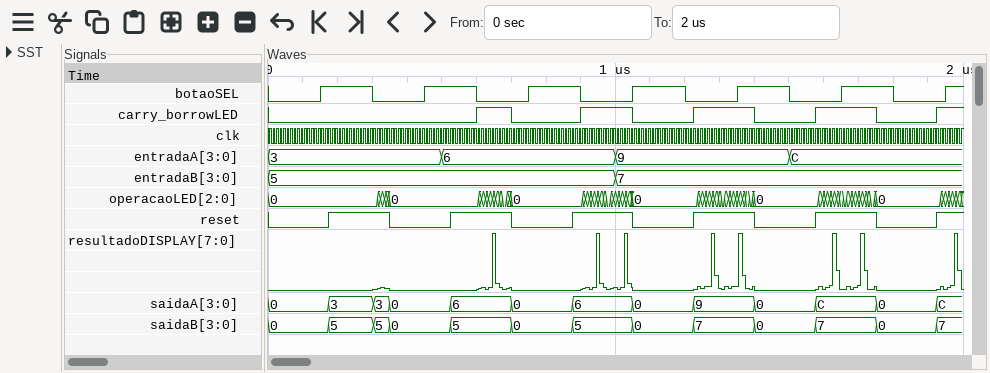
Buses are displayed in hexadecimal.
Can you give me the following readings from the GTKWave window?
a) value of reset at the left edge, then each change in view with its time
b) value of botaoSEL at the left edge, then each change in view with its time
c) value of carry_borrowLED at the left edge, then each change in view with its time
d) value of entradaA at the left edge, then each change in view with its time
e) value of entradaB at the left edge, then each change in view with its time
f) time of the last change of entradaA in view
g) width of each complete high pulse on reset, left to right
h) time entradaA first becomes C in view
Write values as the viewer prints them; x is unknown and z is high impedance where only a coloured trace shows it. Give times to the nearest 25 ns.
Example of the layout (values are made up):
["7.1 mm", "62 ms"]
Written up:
["0, 1 at 175 ns, 0 at 350 ns, 1 at 525 ns, 0 at 700 ns, 1 at 875 ns, 0 at 1050 ns, 1 at 1225 ns, 0 at 1400 ns, 1 at 1575 ns, 0 at 1750 ns, 1 at 1925 ns", "0, 1 at 150 ns, 0 at 300 ns, 1 at 450 ns, 0 at 600 ns, 1 at 750 ns, 0 at 900 ns, 1 at 1050 ns, 0 at 1200 ns, 1 at 1350 ns, 0 at 1500 ns, 1 at 1650 ns, 0 at 1800 ns, 1 at 1950 ns", "0, 1 at 600 ns, 0 at 700 ns, 1 at 900 ns, 0 at 1050 ns, 1 at 1225 ns, 0 at 1400 ns, 1 at 1575 ns, 0 at 1750 ns, 1 at 1925 ns", "3, 6 at 500 ns, 9 at 1000 ns, C at 1500 ns", "5, 7 at 1000 ns", "1500 ns", "175 ns, 175 ns, 175 ns, 175 ns, 175 ns", "1500 ns"]
